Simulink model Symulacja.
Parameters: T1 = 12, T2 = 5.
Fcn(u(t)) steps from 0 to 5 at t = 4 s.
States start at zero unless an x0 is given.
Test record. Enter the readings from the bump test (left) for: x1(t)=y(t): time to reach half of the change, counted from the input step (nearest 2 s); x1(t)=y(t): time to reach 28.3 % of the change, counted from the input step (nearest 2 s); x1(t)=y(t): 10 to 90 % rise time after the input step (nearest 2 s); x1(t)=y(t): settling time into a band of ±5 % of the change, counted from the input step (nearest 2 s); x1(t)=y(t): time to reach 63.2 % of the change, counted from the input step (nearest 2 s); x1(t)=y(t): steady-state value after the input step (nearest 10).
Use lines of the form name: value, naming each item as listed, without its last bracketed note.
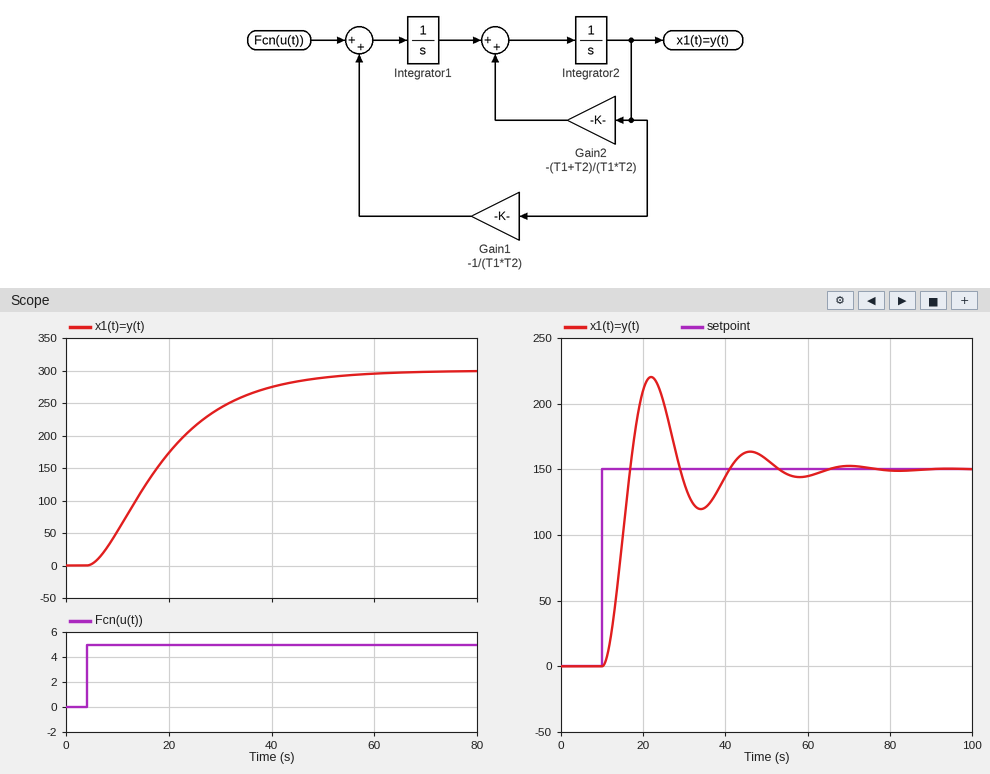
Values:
x1(t)=y(t): time to reach half of the change, counted from the input step: 14 s
x1(t)=y(t): time to reach 28.3 % of the change, counted from the input step: 8 s
x1(t)=y(t): 10 to 90 % rise time after the input step: 30 s
x1(t)=y(t): settling time into a band of ±5 % of the change, counted from the input step: 42 s
x1(t)=y(t): time to reach 63.2 % of the change, counted from the input step: 18 s
x1(t)=y(t): steady-state value after the input step: 300
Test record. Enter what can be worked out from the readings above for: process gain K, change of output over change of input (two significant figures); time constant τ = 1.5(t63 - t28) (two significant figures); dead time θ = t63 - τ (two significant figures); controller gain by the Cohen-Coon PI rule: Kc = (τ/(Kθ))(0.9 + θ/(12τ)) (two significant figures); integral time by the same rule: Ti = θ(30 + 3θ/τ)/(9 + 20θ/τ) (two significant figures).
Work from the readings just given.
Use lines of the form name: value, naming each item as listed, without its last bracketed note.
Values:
process gain K, change of output over change of input: 60
time constant τ = 1.5(t63 - t28): 15 s
dead time θ = t63 - τ: 3.0 s
controller gain by the Cohen-Coon PI rule: Kc = (τ/(Kθ))(0.9 + θ/(12τ)): 0.076
integral time by the same rule: Ti = θ(30 + 3θ/τ)/(9 + 20θ/τ): 7.1 s
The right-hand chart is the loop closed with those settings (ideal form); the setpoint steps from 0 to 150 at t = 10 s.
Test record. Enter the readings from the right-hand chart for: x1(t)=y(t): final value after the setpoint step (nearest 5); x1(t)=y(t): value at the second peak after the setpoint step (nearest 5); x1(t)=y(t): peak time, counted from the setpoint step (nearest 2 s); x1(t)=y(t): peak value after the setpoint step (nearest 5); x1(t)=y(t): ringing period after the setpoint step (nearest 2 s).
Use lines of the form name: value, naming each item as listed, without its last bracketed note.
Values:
x1(t)=y(t): final value after the setpoint step: 150
x1(t)=y(t): value at the second peak after the setpoint step: 165
x1(t)=y(t): peak time, counted from the setpoint step: 12 s
x1(t)=y(t): peak value after the setpoint step: 220
x1(t)=y(t): ringing period after the setpoint step: 24 s
